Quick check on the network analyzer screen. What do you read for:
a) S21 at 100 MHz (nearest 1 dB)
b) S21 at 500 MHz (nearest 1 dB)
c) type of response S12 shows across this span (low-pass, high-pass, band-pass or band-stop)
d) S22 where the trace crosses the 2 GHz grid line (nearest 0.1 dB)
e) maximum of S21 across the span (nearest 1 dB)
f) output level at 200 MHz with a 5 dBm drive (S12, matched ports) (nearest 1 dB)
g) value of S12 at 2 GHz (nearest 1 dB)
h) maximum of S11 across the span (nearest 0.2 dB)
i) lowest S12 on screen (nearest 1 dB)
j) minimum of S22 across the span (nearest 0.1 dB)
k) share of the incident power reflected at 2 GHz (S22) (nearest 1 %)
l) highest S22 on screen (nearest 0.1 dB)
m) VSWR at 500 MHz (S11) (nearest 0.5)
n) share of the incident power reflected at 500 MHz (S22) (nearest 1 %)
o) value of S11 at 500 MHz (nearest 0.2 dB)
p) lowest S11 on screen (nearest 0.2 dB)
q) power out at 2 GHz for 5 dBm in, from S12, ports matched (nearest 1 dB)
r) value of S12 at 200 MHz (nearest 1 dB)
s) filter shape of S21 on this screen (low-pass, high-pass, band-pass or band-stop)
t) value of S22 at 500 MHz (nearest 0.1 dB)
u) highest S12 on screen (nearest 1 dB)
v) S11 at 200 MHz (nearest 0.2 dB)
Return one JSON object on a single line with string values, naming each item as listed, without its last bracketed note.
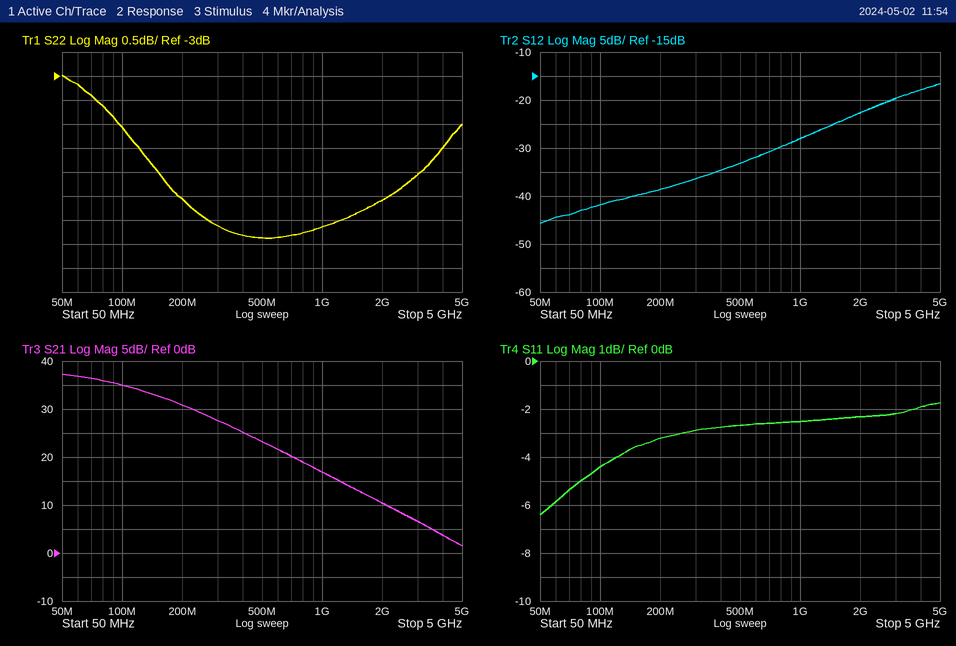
{"S21 at 100 MHz": "35 dB", "S21 at 500 MHz": "23 dB", "type of response S12 shows across this span": "high-pass", "S22 where the trace crosses the 2 GHz grid line": "-5.6 dB", "maximum of S21 across the span": "37 dB", "output level at 200 MHz with a 5 dBm drive (S12, matched ports)": "-34 dBm", "value of S12 at 2 GHz": "-23 dB", "maximum of S11 across the span": "-1.8 dB", "lowest S12 on screen": "-46 dB", "minimum of S22 across the span": "-6.4 dB", "share of the incident power reflected at 2 GHz (S22)": "28 %", "highest S22 on screen": "-3.0 dB", "VSWR at 500 MHz (S11)": "6.5", "share of the incident power reflected at 500 MHz (S22)": "23 %", "value of S11 at 500 MHz": "-2.6 dB", "lowest S11 on screen": "-6.4 dB", "power out at 2 GHz for 5 dBm in, from S12, ports matched": "-18 dBm", "value of S12 at 200 MHz": "-39 dB", "filter shape of S21 on this screen": "low-pass", "value of S22 at 500 MHz": "-6.4 dB", "highest S12 on screen": "-17 dB", "S11 at 200 MHz": "-3.2 dB"}
